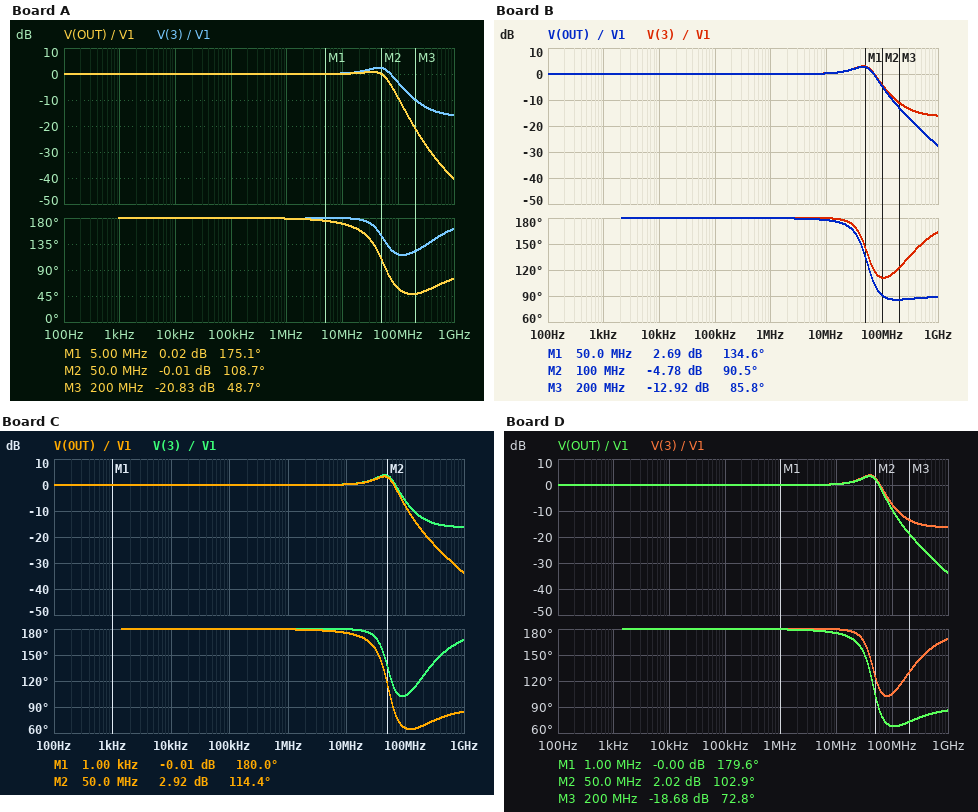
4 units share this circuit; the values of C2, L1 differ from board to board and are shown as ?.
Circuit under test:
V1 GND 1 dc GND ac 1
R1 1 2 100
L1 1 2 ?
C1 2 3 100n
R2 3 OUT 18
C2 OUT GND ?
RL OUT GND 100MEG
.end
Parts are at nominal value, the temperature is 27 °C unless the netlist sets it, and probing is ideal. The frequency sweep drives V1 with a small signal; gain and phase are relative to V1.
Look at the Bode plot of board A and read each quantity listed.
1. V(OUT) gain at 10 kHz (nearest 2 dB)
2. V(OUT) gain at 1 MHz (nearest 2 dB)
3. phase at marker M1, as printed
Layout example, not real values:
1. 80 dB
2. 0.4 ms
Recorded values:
1. 0 dB
2. 0 dB
3. 175.1 deg
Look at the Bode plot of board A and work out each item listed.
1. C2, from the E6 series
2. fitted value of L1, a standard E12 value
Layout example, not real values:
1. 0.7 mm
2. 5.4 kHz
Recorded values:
1. 150 pF
2. 47 nH
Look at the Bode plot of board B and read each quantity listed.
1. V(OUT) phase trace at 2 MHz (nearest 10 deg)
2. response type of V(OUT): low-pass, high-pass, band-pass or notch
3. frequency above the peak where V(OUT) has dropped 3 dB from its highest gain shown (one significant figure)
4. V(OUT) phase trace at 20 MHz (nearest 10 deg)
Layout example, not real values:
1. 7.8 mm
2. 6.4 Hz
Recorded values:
1. 180 deg
2. low-pass
3. 70 MHz
4. 170 deg
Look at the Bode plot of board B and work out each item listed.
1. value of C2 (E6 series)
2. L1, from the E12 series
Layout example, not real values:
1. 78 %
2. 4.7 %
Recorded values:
1. 33 pF
2. 220 nH
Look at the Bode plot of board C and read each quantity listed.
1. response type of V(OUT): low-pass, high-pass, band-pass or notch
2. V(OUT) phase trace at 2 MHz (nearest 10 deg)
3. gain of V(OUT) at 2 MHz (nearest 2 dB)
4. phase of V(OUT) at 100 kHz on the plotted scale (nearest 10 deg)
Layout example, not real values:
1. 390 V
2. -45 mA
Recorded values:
1. low-pass
2. 180 deg
3. 0 dB
4. 180 deg
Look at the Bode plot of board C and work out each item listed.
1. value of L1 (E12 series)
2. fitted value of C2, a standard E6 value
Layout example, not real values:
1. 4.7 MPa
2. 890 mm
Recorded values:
1. 120 nH
2. 68 pF
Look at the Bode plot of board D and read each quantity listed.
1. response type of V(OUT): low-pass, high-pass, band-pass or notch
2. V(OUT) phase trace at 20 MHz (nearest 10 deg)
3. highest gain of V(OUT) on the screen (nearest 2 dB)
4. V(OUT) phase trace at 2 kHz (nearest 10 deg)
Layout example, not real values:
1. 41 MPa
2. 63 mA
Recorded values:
1. low-pass
2. 170 deg
3. 4 dB
4. 180 deg
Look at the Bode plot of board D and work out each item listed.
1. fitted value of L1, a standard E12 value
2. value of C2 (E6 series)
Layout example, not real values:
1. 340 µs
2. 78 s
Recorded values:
1. 150 nH
2. 68 pF
